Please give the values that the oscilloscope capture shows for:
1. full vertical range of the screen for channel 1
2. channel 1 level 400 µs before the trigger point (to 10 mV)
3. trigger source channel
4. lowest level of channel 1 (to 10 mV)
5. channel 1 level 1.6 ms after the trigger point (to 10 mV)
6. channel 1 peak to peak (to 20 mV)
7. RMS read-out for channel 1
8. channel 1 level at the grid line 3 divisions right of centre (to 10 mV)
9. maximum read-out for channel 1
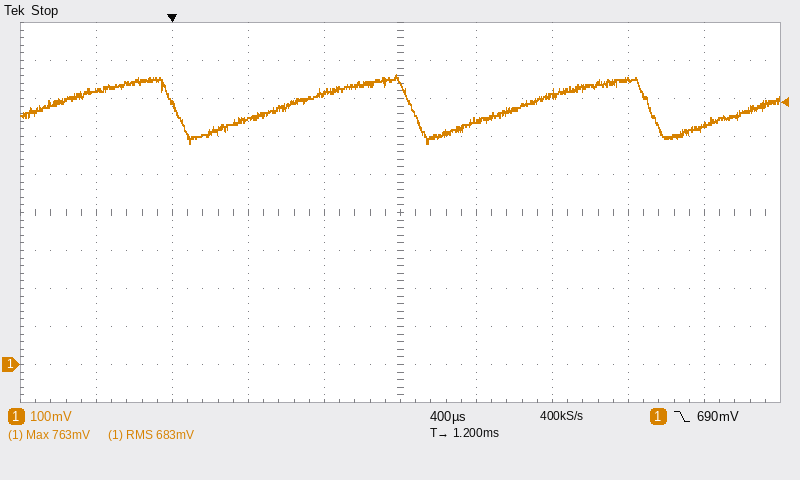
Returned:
1 V
720 mV
channel 1
580 mV
640 mV
180 mV
683 mV
750 mV
763 mV
